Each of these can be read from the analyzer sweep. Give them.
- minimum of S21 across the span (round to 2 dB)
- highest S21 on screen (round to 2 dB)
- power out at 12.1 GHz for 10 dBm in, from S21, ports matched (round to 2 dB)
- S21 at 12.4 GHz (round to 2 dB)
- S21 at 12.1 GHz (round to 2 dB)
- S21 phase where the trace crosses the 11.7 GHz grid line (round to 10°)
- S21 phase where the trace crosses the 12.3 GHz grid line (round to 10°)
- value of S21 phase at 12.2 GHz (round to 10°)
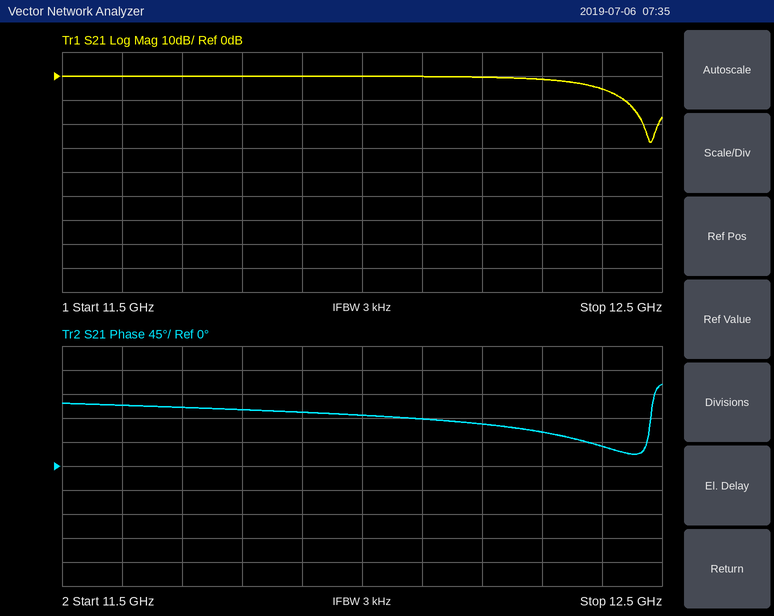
-28 dB
0 dB
10 dBm
-6 dB
0 dB
110°
60°
80°
